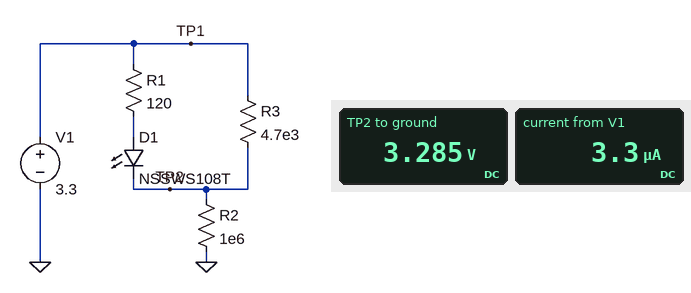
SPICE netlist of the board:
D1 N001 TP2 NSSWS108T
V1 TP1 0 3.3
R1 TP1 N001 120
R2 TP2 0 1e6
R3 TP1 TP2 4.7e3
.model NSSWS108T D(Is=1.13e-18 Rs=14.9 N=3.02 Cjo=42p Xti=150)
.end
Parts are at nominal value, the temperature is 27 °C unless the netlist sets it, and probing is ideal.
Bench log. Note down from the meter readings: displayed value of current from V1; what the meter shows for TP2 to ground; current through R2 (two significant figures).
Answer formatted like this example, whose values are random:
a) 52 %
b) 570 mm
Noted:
a) 3.3 µA
b) 3.285 V
c) 3.3 µA
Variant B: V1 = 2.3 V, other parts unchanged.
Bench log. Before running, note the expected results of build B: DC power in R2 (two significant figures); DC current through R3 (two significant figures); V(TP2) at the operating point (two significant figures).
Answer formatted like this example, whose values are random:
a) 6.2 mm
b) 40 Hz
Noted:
a) 5.2 µW
b) 2.3 µA
c) 2.3 V
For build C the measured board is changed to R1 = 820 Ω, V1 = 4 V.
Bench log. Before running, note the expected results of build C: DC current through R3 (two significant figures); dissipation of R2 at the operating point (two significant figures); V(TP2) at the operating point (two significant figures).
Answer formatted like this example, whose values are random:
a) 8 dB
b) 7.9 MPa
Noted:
a) 4.0 µA
b) 16 µW
c) 4.0 V
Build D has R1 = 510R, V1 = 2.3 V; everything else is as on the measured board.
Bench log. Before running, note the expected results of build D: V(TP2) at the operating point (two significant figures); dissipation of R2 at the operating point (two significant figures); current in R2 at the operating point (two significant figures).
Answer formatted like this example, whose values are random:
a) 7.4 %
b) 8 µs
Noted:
a) 2.3 V
b) 5.2 µW
c) 2.3 µA
